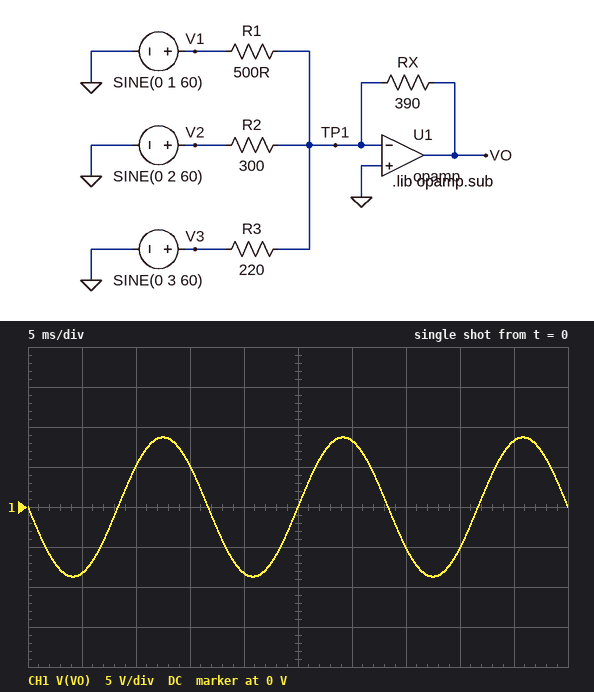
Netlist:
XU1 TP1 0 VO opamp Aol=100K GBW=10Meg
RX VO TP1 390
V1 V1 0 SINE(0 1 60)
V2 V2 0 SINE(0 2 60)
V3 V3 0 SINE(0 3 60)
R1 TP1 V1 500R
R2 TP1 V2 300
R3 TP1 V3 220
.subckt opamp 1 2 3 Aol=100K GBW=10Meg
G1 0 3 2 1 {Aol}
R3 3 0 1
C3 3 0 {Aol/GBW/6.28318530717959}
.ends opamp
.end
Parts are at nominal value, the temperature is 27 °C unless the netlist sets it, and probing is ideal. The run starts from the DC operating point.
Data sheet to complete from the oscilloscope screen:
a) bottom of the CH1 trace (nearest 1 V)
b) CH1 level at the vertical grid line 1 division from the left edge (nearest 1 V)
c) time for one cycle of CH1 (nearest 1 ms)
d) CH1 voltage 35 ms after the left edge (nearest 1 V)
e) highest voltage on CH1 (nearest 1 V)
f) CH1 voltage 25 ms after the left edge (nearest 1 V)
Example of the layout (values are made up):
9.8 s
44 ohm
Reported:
-9 V
-8 V
17 ms
-5 V
9 V
0 V
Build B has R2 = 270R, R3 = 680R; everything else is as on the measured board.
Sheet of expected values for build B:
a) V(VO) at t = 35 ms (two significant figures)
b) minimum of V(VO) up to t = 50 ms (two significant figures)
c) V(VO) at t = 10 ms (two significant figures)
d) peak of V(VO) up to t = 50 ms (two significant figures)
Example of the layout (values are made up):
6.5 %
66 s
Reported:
-3.2 V
-5.4 V
3.2 V
5.4 V
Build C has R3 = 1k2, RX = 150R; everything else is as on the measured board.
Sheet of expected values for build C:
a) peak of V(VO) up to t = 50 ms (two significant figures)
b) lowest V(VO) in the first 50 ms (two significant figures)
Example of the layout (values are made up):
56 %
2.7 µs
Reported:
1.7 V
-1.7 V
